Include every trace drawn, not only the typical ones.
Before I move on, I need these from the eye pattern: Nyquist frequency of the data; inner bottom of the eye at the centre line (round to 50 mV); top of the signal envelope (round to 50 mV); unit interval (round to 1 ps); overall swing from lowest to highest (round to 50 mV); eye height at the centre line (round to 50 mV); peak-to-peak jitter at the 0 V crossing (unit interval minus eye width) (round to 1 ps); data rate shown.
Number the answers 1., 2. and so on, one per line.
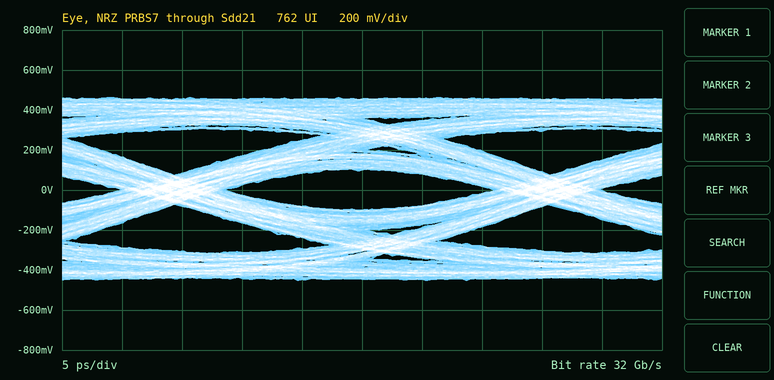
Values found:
1. 16 GHz
2. -100 mV
3. 450 mV
4. 31 ps
5. 900 mV
6. 200 mV
7. 9 ps
8. 32 Gb/s
